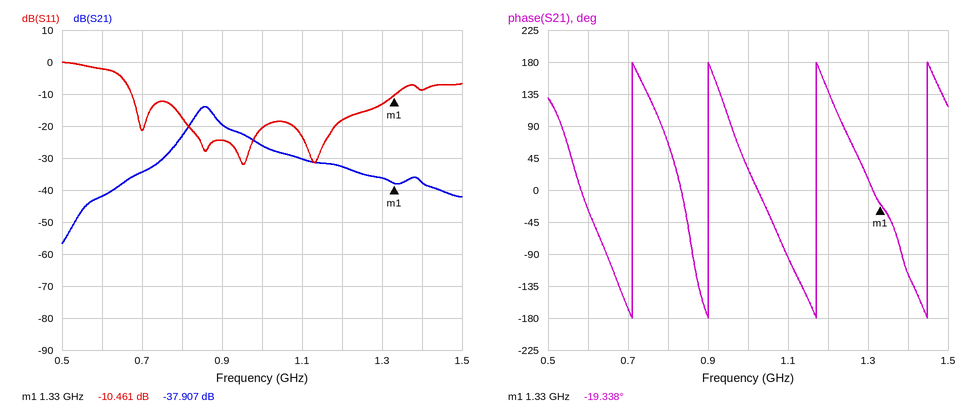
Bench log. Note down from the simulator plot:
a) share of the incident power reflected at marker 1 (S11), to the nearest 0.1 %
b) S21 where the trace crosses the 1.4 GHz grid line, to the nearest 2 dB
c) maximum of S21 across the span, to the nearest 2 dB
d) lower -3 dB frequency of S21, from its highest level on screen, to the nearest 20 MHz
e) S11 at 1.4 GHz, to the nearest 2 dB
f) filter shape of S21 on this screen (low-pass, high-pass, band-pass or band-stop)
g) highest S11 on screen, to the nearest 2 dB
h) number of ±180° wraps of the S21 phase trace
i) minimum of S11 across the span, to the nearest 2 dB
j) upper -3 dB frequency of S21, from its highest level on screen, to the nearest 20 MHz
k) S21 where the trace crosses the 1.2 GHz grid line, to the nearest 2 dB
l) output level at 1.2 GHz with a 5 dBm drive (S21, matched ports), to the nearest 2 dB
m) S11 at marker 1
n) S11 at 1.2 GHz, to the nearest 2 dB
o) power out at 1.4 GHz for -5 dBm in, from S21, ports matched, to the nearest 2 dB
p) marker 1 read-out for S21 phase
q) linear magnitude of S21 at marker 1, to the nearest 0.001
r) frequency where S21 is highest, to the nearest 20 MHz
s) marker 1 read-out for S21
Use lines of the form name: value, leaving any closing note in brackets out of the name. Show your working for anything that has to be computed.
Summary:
share of the incident power reflected at marker 1 (S11), to the nearest 0.1 %: 10^(-10.461/10) ≈ 9.0 %
S21 where the trace crosses the 1.4 GHz grid line, to the nearest 2 dB: -38 dB
maximum of S21 across the span, to the nearest 2 dB: -14 dB
lower -3 dB frequency of S21, from its highest level on screen, to the nearest 20 MHz: 840 MHz
S11 at 1.4 GHz, to the nearest 2 dB: -8 dB
filter shape of S21 on this screen: band-pass
highest S11 on screen, to the nearest 2 dB: 0 dB
number of ±180° wraps of the S21 phase trace: 4
minimum of S11 across the span, to the nearest 2 dB: -32 dB
upper -3 dB frequency of S21, from its highest level on screen, to the nearest 20 MHz: 880 MHz
S21 where the trace crosses the 1.2 GHz grid line, to the nearest 2 dB: -32 dB
output level at 1.2 GHz with a 5 dBm drive (S21, matched ports), to the nearest 2 dB: 5 dBm + (-32 dB) = -28 dBm
S11 at marker 1: -10.461 dB
S11 at 1.2 GHz, to the nearest 2 dB: -18 dB
power out at 1.4 GHz for -5 dBm in, from S21, ports matched, to the nearest 2 dB: -5 dBm + (-38 dB) = -42 dBm
marker 1 read-out for S21 phase: -19.338°
linear magnitude of S21 at marker 1, to the nearest 0.001: 10^(-37.907/20) ≈ 0.013
frequency where S21 is highest, to the nearest 20 MHz: 860 MHz
marker 1 read-out for S21: -37.907 dB
